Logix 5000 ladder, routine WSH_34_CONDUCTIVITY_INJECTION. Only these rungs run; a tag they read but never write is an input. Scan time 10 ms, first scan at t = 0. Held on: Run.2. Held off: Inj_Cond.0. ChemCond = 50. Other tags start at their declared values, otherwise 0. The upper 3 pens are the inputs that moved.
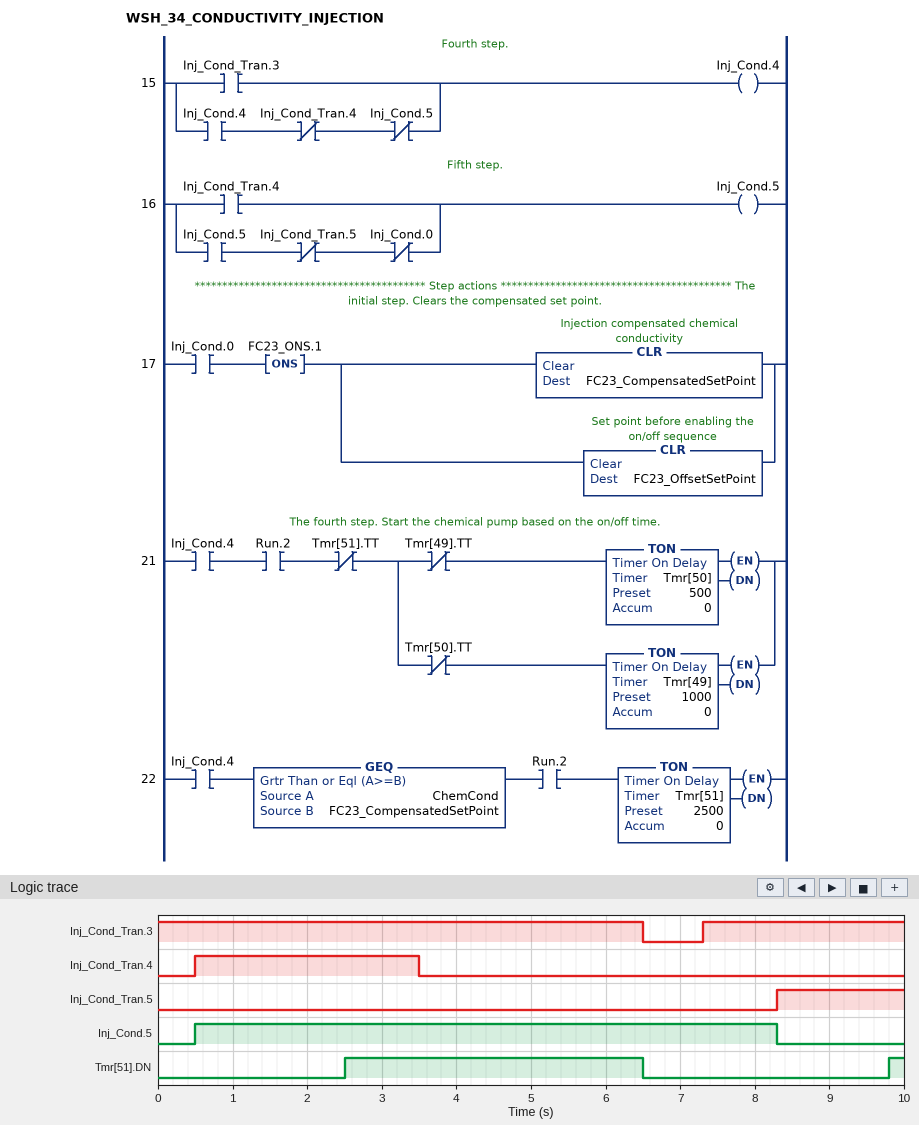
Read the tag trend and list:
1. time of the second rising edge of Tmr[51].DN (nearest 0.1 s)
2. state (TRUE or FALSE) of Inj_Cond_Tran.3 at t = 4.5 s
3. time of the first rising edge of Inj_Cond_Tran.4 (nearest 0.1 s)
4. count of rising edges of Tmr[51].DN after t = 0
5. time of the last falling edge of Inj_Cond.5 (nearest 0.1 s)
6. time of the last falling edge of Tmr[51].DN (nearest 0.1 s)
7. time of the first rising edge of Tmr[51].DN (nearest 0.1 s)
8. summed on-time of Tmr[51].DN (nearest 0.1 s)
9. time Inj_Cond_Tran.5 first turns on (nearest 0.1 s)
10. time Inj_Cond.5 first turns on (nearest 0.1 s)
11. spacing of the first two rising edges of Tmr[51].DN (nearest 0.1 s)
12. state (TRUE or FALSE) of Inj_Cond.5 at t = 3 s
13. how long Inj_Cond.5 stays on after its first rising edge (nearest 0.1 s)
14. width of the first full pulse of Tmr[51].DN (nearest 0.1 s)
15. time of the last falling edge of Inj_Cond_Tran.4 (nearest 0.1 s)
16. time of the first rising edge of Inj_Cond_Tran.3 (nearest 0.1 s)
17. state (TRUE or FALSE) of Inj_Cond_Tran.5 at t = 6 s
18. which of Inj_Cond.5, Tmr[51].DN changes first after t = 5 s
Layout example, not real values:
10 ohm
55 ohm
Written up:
9.8 s
TRUE
0.5 s
2
8.3 s
6.5 s
2.5 s
4.2 s
8.3 s
0.5 s
7.3 s
TRUE
7.8 s
4.0 s
3.5 s
7.3 s
FALSE
Tmr[51].DN
